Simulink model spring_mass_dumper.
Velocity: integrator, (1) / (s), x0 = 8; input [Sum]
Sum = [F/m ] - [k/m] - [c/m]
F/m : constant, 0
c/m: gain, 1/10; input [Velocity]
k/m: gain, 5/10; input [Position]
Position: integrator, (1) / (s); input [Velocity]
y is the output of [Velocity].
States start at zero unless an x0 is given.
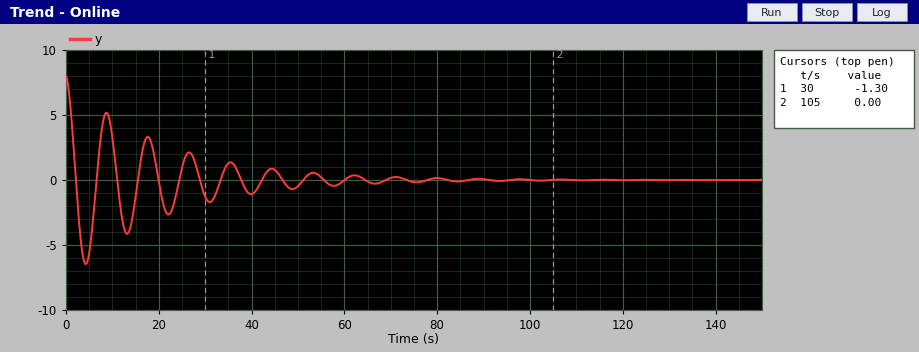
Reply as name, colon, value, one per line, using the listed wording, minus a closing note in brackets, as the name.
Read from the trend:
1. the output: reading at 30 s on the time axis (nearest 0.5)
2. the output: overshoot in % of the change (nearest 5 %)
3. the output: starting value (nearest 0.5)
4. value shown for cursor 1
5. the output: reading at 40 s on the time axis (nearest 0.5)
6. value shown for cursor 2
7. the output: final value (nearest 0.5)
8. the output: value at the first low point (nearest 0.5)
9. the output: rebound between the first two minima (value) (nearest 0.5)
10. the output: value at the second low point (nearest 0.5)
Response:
the output: reading at 30 s on the time axis: -1.5
the output: overshoot in % of the change: 80 %
the output: starting value: 8.0
value shown for cursor 1: -1.30
the output: reading at 40 s on the time axis: -1.0
value shown for cursor 2: 0.00
the output: final value: 0.0
the output: value at the first low point: -6.5
the output: rebound between the first two minima (value): 5.0
the output: value at the second low point: -4.0
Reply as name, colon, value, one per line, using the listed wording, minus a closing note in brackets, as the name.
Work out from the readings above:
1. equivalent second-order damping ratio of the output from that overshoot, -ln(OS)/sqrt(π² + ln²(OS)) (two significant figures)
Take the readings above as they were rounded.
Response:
equivalent second-order damping ratio of the output from that overshoot, -ln(OS)/sqrt(π² + ln²(OS)): 0.071
